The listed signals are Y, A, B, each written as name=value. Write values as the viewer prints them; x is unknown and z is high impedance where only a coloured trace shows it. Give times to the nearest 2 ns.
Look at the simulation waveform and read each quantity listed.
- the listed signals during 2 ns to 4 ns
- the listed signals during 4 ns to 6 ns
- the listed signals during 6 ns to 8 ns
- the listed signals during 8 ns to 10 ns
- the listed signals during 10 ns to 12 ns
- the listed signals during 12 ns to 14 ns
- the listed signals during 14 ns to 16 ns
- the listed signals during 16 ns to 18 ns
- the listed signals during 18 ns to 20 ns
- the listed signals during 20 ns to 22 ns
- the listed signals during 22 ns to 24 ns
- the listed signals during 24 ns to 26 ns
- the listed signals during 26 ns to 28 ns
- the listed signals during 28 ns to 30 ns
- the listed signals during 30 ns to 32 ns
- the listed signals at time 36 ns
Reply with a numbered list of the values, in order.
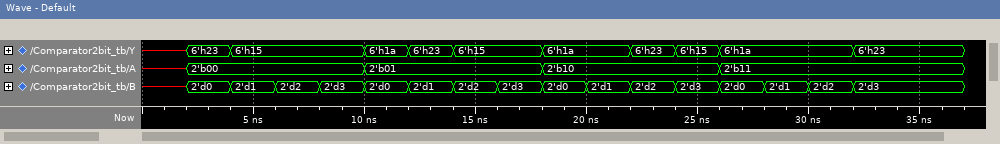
1. Y=6'h23, A=2'b00, B=2'd0
2. Y=6'h15, A=2'b00, B=2'd1
3. Y=6'h15, A=2'b00, B=2'd2
4. Y=6'h15, A=2'b00, B=2'd3
5. Y=6'h1a, A=2'b01, B=2'd0
6. Y=6'h23, A=2'b01, B=2'd1
7. Y=6'h15, A=2'b01, B=2'd2
8. Y=6'h15, A=2'b01, B=2'd3
9. Y=6'h1a, A=2'b10, B=2'd0
10. Y=6'h1a, A=2'b10, B=2'd1
11. Y=6'h23, A=2'b10, B=2'd2
12. Y=6'h15, A=2'b10, B=2'd3
13. Y=6'h1a, A=2'b11, B=2'd0
14. Y=6'h1a, A=2'b11, B=2'd1
15. Y=6'h1a, A=2'b11, B=2'd2
16. Y=6'h23, A=2'b11, B=2'd3
